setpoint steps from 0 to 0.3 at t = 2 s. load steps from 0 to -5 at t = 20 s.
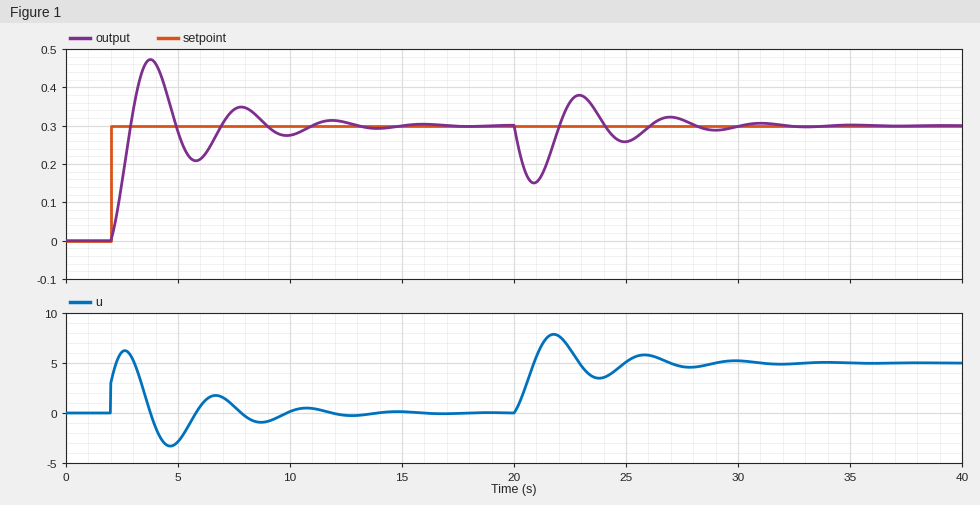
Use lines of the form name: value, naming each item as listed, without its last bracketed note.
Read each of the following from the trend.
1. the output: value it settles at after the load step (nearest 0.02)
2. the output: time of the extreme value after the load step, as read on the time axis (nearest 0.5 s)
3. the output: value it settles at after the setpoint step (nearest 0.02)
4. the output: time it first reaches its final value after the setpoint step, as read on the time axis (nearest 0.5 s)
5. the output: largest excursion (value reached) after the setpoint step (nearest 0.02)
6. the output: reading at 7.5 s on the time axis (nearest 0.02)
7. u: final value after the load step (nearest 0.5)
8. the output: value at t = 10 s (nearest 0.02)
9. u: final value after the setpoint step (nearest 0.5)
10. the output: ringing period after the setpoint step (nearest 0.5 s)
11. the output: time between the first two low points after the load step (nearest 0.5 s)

the output: value it settles at after the load step: 0.30
the output: time of the extreme value after the load step, as read on the time axis: 21.0 s
the output: value it settles at after the setpoint step: 0.30
the output: time it first reaches its final value after the setpoint step, as read on the time axis: 3.0 s
the output: largest excursion (value reached) after the setpoint step: 0.48
the output: reading at 7.5 s on the time axis: 0.34
u: final value after the load step: 5.0
the output: value at t = 10 s: 0.28
u: final value after the setpoint step: 0.0
the output: ringing period after the setpoint step: 4.0 s
the output: time between the first two low points after the load step: 4.0 s
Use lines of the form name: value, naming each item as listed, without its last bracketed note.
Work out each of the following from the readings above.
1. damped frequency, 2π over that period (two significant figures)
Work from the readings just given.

damped frequency, 2π over that period: 1.6 rad/s
